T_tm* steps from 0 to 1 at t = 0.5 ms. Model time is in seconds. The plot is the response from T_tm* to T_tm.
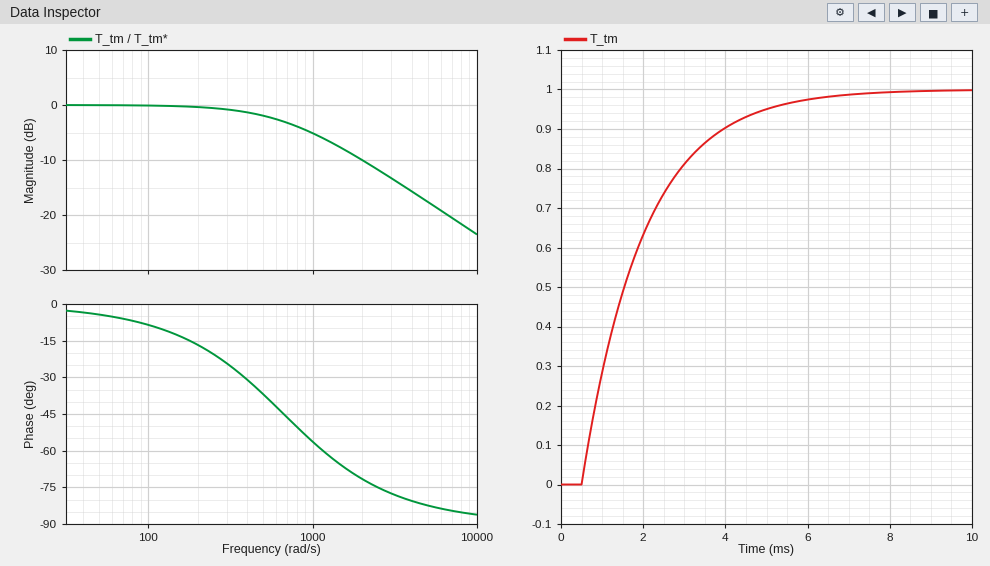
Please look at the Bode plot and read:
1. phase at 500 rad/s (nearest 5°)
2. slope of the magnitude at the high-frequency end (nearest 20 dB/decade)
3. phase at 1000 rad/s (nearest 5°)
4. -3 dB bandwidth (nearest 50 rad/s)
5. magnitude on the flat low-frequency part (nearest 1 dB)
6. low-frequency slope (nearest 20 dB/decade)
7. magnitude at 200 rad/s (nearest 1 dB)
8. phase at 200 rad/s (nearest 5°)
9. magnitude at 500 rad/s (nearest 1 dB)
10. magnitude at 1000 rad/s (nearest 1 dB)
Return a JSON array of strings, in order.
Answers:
["-35°", "-20 dB/decade", "-55°", "650 rad/s", "0 dB", "0 dB/decade", "0 dB", "-15°", "-2 dB", "-5 dB"]
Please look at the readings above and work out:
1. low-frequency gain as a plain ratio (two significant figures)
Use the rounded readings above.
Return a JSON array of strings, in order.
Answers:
["1.0"]
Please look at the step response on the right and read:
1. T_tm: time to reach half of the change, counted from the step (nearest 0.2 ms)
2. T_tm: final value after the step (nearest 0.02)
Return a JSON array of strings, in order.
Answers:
["1.0 ms", "1.00"]
